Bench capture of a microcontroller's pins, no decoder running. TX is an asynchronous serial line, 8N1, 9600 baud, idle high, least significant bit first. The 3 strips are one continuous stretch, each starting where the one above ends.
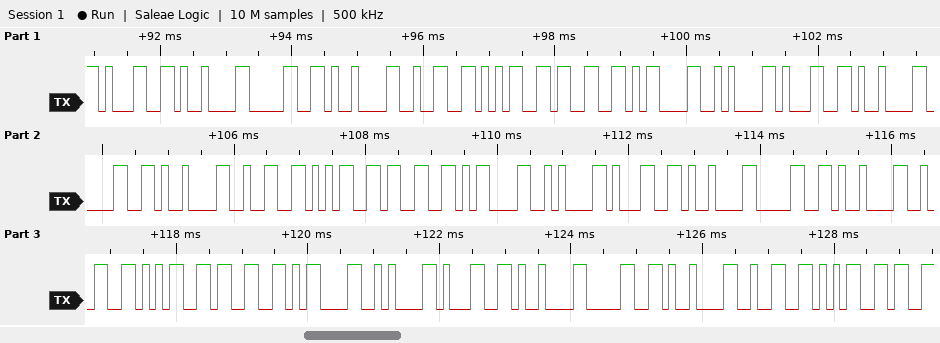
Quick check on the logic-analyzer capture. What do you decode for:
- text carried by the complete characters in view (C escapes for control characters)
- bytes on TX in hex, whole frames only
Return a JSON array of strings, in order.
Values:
["\"1\\t0\\t253\\r\\n1\\t0\\t253\\r\\n1\\t0\\t253\\r\\n1\\t0\\t25\"", "0x31 0x09 0x30 0x09 0x32 0x35 0x33 0x0D 0x0A 0x31 0x09 0x30 0x09 0x32 0x35 0x33 0x0D 0x0A 0x31 0x09 0x30 0x09 0x32 0x35 0x33 0x0D 0x0A 0x31 0x09 0x30 0x09 0x32 0x35"]
